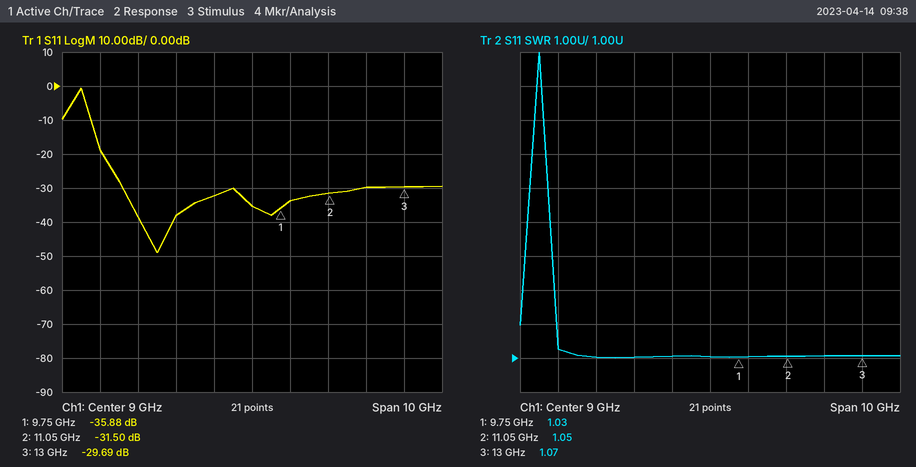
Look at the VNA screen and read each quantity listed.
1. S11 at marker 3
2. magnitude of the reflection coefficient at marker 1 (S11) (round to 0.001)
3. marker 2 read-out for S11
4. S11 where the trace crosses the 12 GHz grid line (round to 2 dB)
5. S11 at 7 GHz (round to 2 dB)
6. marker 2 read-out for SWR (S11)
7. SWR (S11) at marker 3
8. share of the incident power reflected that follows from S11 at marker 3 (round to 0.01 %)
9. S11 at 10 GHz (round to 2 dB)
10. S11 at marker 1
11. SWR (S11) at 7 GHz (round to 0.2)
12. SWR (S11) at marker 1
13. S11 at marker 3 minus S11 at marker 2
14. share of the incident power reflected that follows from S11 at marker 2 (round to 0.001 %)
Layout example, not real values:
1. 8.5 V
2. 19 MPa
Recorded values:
1. -29.69 dB
2. 0.016
3. -31.50 dB
4. -30 dB
5. -38 dB
6. 1.05
7. 1.07
8. 0.11 %
9. -34 dB
10. -35.88 dB
11. 1.0
12. 1.03
13. 1.81 dB
14. 0.071 %
